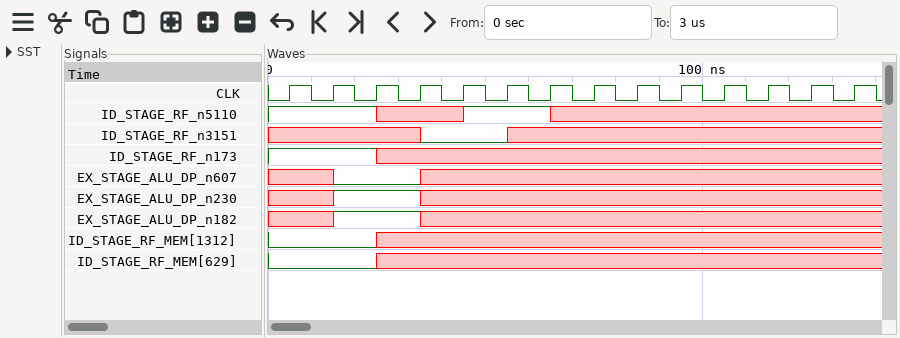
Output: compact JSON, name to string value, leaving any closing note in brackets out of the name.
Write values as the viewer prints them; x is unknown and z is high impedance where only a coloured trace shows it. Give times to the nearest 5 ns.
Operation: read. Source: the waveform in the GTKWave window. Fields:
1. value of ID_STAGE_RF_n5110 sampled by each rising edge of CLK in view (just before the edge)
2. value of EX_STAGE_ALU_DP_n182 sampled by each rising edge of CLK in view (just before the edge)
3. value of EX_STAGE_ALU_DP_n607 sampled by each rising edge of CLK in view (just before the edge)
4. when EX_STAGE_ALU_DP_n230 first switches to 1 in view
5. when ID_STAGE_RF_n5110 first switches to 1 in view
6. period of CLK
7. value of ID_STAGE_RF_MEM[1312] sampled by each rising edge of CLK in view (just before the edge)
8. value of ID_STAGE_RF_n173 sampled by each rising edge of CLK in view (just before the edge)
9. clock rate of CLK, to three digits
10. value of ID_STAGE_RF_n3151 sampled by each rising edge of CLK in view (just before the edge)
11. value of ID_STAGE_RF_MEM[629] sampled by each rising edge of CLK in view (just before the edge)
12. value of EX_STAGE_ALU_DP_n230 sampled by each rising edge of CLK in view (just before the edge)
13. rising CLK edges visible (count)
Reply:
{"value of ID_STAGE_RF_n5110 sampled by each rising edge of CLK in view": "1 1 1 x x 1 1 x x x x x x x", "value of EX_STAGE_ALU_DP_n182 sampled by each rising edge of CLK in view": "x x 1 1 x x x x x x x x x x", "value of EX_STAGE_ALU_DP_n607 sampled by each rising edge of CLK in view": "x x 0 0 x x x x x x x x x x", "when EX_STAGE_ALU_DP_n230 first switches to 1 in view": "15 ns", "when ID_STAGE_RF_n5110 first switches to 1 in view": "45 ns", "period of CLK": "10 ns", "value of ID_STAGE_RF_MEM[1312] sampled by each rising edge of CLK in view": "0 0 0 x x x x x x x x x x x", "value of ID_STAGE_RF_n173 sampled by each rising edge of CLK in view": "1 1 1 x x x x x x x x x x x", "clock rate of CLK, to three digits": "100 MHz", "value of ID_STAGE_RF_n3151 sampled by each rising edge of CLK in view": "x x x x 0 0 x x x x x x x x", "value of ID_STAGE_RF_MEM[629] sampled by each rising edge of CLK in view": "0 0 0 x x x x x x x x x x x", "value of EX_STAGE_ALU_DP_n230 sampled by each rising edge of CLK in view": "x x 1 1 x x x x x x x x x x", "rising CLK edges visible": "14"}
